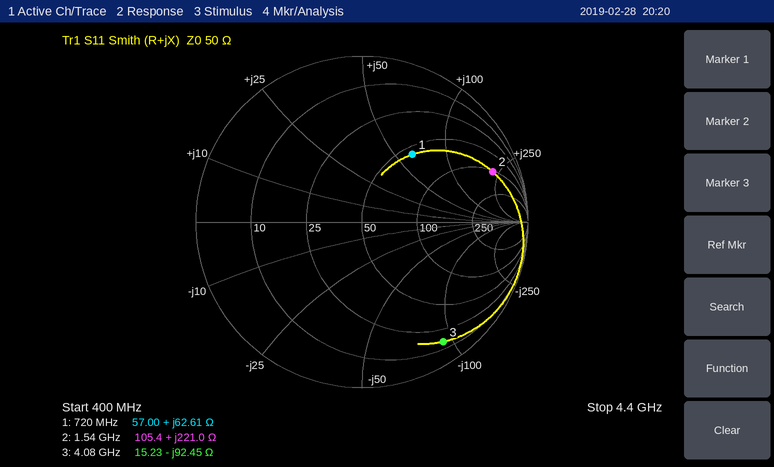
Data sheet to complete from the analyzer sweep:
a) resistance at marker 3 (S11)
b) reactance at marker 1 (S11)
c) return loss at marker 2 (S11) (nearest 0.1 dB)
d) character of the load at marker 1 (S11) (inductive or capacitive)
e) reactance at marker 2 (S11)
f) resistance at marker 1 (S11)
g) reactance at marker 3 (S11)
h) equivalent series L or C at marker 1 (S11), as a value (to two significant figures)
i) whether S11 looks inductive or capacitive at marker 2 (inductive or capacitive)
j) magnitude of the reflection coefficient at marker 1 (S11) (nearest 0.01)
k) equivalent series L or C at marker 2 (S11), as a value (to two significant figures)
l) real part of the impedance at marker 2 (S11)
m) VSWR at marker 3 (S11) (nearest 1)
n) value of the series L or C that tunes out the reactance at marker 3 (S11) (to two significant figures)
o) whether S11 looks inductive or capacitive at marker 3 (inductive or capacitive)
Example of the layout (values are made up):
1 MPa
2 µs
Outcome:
15.23 Ω
+62.61 Ω
1.5 dB
inductive
+221.0 Ω
57.00 Ω
-92.45 Ω
14 nH
inductive
0.51
23 nH
105.4 Ω
15
3.6 nH
capacitive
